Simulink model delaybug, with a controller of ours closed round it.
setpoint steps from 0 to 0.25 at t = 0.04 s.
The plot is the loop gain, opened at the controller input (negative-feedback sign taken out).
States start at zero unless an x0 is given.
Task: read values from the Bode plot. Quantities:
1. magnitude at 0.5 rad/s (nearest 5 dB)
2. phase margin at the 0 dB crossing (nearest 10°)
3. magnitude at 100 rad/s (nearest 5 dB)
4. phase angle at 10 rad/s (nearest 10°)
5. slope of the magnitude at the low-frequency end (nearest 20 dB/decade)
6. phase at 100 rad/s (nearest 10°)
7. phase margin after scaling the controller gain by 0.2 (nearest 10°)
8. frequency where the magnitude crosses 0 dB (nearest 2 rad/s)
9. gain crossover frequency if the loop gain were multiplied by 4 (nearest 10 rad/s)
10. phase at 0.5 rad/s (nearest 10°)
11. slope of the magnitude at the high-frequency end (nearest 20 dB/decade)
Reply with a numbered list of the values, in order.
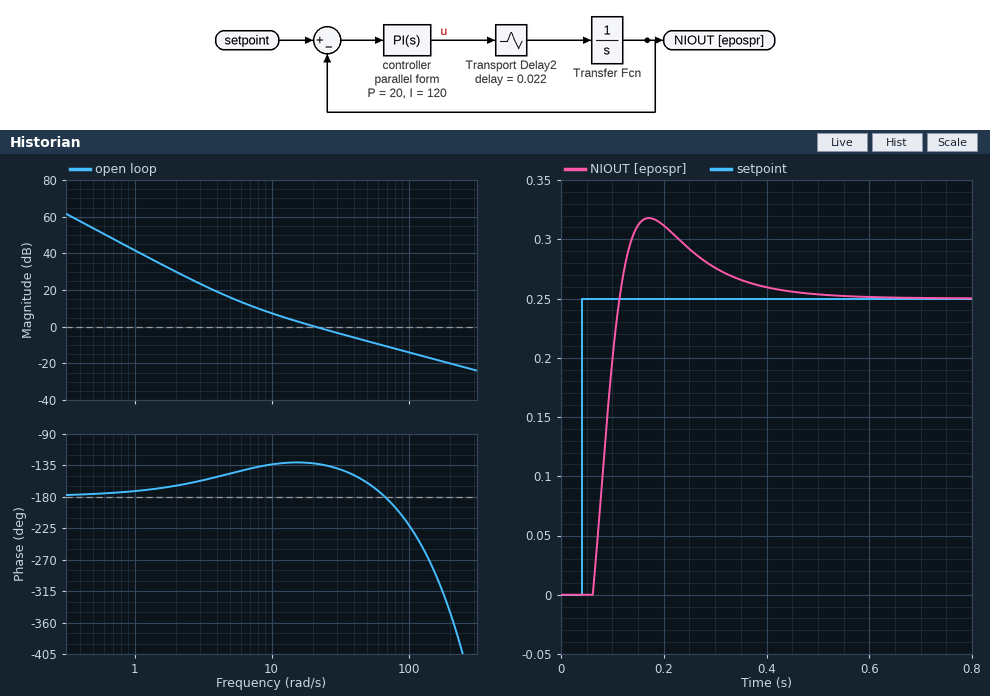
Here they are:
1. 55 dB
2. 50°
3. -15 dB
4. -130°
5. -40 dB/decade
6. -220°
7. 40°
8. 20 rad/s
9. 80 rad/s
10. -180°
11. -20 dB/decade
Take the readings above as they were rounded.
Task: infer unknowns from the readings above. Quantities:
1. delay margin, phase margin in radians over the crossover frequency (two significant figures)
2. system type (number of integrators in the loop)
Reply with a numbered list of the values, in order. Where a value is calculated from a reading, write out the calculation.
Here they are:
1. 50 × π / 180 / 20 = 0.044 s
2. 2
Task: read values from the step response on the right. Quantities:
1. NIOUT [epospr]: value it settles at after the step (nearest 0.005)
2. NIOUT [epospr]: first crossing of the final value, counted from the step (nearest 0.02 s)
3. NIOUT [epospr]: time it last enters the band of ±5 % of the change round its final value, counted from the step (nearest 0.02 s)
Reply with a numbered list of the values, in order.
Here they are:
1. 0.250
2. 0.08 s
3. 0.34 s
